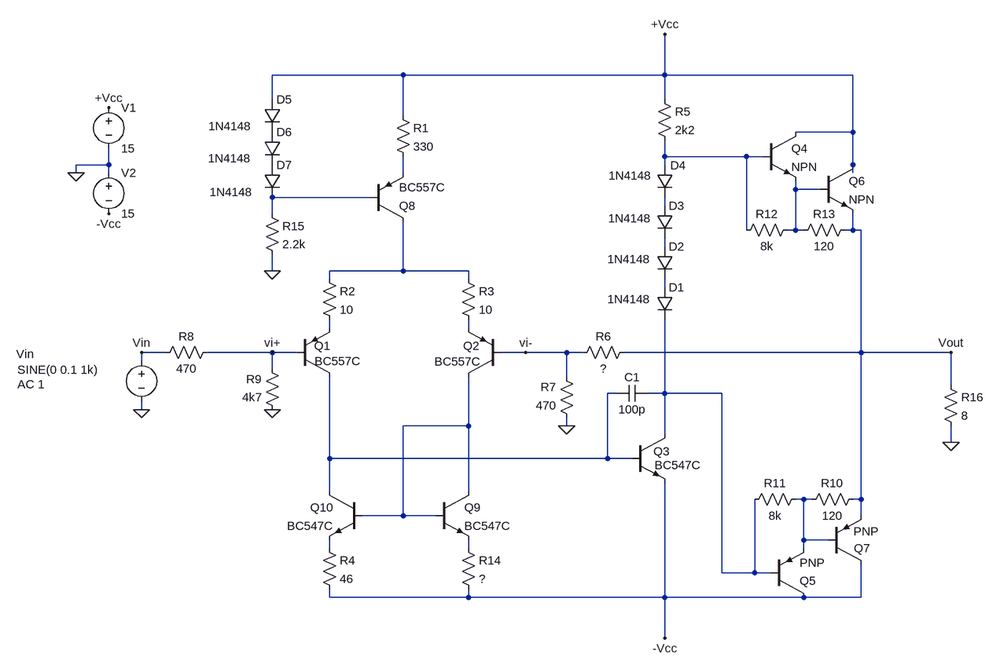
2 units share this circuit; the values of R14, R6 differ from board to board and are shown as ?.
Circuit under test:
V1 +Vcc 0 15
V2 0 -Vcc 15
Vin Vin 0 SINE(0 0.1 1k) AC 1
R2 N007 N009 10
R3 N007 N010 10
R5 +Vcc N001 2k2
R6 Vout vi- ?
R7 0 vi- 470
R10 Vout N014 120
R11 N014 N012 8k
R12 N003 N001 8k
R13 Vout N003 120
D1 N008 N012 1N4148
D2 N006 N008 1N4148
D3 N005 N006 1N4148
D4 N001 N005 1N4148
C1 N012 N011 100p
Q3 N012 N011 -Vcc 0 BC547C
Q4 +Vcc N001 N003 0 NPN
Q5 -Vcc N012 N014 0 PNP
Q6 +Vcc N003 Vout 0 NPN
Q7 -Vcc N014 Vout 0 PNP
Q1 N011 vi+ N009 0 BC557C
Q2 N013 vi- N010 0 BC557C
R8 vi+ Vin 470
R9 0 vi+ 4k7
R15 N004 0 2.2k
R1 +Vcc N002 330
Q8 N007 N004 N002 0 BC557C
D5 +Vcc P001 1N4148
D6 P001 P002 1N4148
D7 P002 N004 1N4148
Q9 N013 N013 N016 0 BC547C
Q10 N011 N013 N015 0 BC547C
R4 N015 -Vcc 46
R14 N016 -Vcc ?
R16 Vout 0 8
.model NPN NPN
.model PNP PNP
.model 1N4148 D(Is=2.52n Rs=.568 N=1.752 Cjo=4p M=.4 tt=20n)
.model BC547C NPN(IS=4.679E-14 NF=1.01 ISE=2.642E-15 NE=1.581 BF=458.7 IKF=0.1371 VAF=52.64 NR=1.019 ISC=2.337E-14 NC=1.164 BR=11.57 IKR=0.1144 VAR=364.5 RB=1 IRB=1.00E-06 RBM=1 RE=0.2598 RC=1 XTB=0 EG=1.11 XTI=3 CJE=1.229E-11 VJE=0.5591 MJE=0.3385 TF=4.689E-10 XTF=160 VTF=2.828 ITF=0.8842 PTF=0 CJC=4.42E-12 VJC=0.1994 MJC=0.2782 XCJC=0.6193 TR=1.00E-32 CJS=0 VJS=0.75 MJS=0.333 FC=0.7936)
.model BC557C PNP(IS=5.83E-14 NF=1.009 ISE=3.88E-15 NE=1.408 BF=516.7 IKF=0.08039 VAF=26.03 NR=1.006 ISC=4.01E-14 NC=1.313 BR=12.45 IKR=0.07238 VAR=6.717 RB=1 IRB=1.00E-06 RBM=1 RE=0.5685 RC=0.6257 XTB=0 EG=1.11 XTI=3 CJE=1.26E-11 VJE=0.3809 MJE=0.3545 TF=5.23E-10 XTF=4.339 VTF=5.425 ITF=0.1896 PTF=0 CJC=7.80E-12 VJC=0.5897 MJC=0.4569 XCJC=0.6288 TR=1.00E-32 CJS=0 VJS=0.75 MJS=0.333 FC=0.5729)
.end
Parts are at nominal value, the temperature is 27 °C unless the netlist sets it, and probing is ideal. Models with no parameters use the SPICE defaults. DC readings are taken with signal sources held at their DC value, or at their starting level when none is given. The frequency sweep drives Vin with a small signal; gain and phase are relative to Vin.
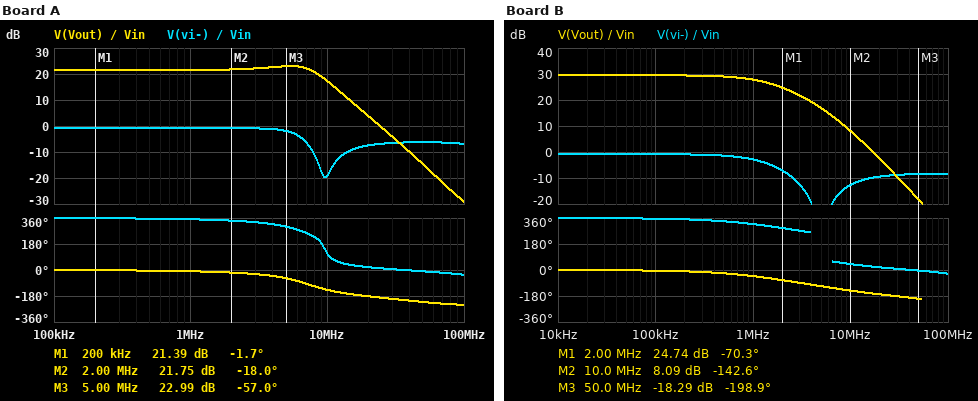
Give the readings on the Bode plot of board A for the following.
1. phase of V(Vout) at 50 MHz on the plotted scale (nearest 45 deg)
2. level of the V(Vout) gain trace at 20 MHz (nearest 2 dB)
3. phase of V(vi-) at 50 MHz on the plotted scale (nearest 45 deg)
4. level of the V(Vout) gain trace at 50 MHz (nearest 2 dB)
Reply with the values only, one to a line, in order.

-225 deg
4 dB
0 deg
-14 dB
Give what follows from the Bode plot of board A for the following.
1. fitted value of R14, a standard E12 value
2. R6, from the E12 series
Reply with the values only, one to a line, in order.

100 Ω
5.6 kΩ
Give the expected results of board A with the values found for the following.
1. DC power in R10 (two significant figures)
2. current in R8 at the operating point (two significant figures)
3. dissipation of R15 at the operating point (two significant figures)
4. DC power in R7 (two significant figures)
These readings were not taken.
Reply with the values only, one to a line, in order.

280 µW
3.4 µA
77 mW
2.2 µW
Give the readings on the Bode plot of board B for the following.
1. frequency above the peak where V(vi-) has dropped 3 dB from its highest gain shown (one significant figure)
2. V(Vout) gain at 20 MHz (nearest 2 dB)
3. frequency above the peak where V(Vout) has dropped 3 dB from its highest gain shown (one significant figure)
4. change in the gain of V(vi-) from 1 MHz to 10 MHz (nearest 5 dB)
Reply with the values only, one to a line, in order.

1 MHz
-2 dB
1 MHz
-10 dB
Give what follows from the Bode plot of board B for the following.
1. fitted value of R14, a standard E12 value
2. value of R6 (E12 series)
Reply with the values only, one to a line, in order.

15 Ω
15 kΩ
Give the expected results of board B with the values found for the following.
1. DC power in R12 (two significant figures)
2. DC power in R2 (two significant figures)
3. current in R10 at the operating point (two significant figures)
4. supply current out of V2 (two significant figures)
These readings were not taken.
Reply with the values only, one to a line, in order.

77 µW
18 µW
7.5 mA
160 mA
